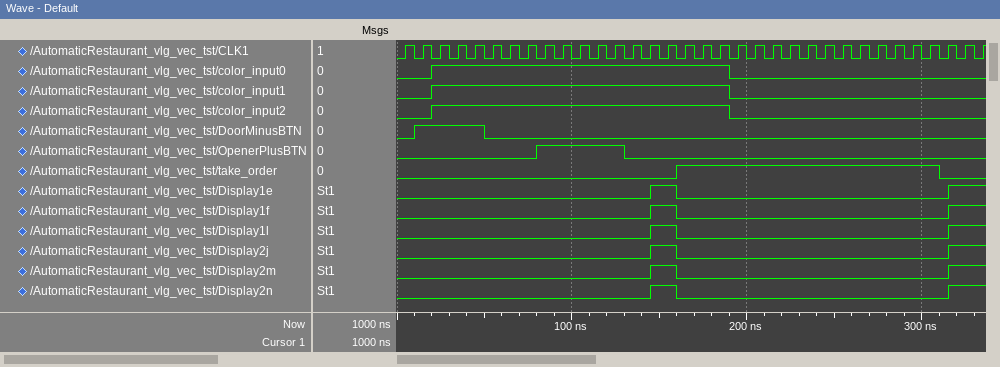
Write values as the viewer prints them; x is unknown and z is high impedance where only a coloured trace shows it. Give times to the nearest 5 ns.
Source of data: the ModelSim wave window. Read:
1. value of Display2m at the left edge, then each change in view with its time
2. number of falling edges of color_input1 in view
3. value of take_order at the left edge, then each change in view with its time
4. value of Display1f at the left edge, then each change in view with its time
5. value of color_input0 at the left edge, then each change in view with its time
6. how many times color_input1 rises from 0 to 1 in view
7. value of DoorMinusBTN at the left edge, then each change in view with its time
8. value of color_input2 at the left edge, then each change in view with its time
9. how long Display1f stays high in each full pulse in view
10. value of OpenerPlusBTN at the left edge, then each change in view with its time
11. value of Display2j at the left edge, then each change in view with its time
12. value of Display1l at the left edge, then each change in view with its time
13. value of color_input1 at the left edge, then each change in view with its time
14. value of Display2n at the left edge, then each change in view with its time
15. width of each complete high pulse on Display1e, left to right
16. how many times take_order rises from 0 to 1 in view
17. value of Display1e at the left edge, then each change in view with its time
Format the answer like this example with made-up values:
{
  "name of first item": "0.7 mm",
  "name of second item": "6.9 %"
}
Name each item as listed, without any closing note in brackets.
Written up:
{
  "value of Display2m at the left edge, then each change in view with its time": "0, 1 at 145 ns, 0 at 160 ns, 1 at 315 ns",
  "number of falling edges of color_input1 in view": "1",
  "value of take_order at the left edge, then each change in view with its time": "0, 1 at 160 ns, 0 at 310 ns",
  "value of Display1f at the left edge, then each change in view with its time": "0, 1 at 145 ns, 0 at 160 ns, 1 at 315 ns",
  "value of color_input0 at the left edge, then each change in view with its time": "0, 1 at 20 ns, 0 at 190 ns",
  "how many times color_input1 rises from 0 to 1 in view": "1",
  "value of DoorMinusBTN at the left edge, then each change in view with its time": "0, 1 at 10 ns, 0 at 50 ns",
  "value of color_input2 at the left edge, then each change in view with its time": "0, 1 at 20 ns, 0 at 190 ns",
  "how long Display1f stays high in each full pulse in view": "15 ns",
  "value of OpenerPlusBTN at the left edge, then each change in view with its time": "0, 1 at 80 ns, 0 at 130 ns",
  "value of Display2j at the left edge, then each change in view with its time": "0, 1 at 145 ns, 0 at 160 ns, 1 at 315 ns",
  "value of Display1l at the left edge, then each change in view with its time": "0, 1 at 145 ns, 0 at 160 ns, 1 at 315 ns",
  "value of color_input1 at the left edge, then each change in view with its time": "0, 1 at 20 ns, 0 at 190 ns",
  "value of Display2n at the left edge, then each change in view with its time": "0, 1 at 145 ns, 0 at 160 ns, 1 at 315 ns",
  "width of each complete high pulse on Display1e, left to right": "15 ns",
  "how many times take_order rises from 0 to 1 in view": "1",
  "value of Display1e at the left edge, then each change in view with its time": "0, 1 at 145 ns, 0 at 160 ns, 1 at 315 ns"
}
